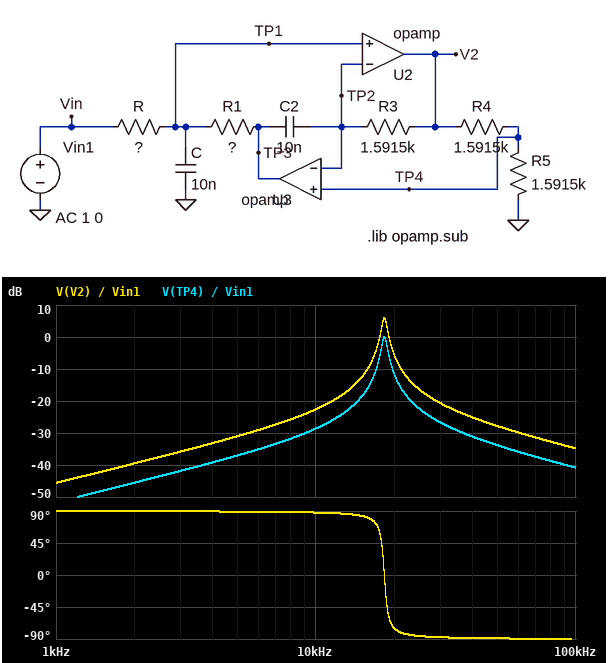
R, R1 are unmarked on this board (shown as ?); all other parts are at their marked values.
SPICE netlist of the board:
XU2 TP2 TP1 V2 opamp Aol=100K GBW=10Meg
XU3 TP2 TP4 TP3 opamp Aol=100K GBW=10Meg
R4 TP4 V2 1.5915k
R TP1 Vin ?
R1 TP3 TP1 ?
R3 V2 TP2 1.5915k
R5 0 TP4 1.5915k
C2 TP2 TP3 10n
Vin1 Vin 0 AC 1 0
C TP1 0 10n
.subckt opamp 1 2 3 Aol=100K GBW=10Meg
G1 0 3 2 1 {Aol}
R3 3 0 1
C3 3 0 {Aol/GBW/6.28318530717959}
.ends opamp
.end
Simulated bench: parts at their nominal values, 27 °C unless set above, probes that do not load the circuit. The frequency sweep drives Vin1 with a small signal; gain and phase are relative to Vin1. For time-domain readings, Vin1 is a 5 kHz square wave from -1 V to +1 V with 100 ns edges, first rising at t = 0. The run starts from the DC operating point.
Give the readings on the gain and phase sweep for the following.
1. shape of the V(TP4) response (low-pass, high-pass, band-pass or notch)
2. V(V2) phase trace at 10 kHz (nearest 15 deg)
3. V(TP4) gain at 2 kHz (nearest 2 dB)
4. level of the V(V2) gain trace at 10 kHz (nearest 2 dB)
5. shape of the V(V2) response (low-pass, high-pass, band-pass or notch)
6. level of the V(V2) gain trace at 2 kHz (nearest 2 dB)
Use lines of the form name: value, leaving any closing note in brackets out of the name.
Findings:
shape of the V(TP4) response: band-pass
V(V2) phase trace at 10 kHz: 90 deg
V(TP4) gain at 2 kHz: -46 dB
level of the V(V2) gain trace at 10 kHz: -22 dB
shape of the V(V2) response: band-pass
level of the V(V2) gain trace at 2 kHz: -40 dB
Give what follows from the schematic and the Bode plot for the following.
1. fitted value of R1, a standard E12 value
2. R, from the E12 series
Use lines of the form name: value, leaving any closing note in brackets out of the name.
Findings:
fitted value of R1, a standard E12 value: 470 Ω
R, from the E12 series: 18 kΩ
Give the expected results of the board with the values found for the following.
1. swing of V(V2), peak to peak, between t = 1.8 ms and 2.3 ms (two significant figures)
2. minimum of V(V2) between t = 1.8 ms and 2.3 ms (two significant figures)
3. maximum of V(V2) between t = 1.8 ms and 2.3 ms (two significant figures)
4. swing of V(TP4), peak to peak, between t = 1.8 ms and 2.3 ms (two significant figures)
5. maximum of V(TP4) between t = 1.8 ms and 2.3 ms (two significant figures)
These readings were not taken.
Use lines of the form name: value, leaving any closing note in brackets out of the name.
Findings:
swing of V(V2), peak to peak, between t = 1.8 ms and 2.3 ms: 250 mV
minimum of V(V2) between t = 1.8 ms and 2.3 ms: -120 mV
maximum of V(V2) between t = 1.8 ms and 2.3 ms: 120 mV
swing of V(TP4), peak to peak, between t = 1.8 ms and 2.3 ms: 120 mV
maximum of V(TP4) between t = 1.8 ms and 2.3 ms: 61 mV
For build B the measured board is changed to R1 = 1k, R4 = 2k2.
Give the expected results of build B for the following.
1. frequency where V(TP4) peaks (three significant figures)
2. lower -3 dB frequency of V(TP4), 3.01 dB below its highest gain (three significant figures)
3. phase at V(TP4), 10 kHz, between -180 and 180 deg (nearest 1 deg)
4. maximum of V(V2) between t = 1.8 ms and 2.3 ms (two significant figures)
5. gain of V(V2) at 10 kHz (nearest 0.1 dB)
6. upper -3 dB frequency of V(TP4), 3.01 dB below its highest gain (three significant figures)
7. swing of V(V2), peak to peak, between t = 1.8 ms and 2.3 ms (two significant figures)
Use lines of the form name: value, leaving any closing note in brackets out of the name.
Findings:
frequency where V(TP4) peaks: 14.8 kHz
lower -3 dB frequency of V(TP4), 3.01 dB below its highest gain: 14.4 kHz
phase at V(TP4), 10 kHz, between -180 and 180 deg: 86 deg
maximum of V(V2) between t = 1.8 ms and 2.3 ms: 1.0 V
gain of V(V2) at 10 kHz: -15.1 dB
upper -3 dB frequency of V(TP4), 3.01 dB below its highest gain: 15.2 kHz
swing of V(V2), peak to peak, between t = 1.8 ms and 2.3 ms: 2.0 V
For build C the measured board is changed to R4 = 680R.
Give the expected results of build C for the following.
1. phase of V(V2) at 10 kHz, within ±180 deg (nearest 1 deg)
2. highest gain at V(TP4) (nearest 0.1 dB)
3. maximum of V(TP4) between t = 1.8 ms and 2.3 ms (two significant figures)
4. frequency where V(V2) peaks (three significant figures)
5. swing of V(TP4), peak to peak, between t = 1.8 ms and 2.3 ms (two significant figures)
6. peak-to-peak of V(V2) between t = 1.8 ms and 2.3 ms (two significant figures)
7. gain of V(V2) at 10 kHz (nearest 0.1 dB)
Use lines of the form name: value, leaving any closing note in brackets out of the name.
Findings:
phase of V(V2) at 10 kHz, within ±180 deg: 78 deg
highest gain at V(TP4): -0.3 dB
maximum of V(TP4) between t = 1.8 ms and 2.3 ms: 95 mV
frequency where V(V2) peaks: 12.0 kHz
swing of V(TP4), peak to peak, between t = 1.8 ms and 2.3 ms: 190 mV
peak-to-peak of V(V2) between t = 1.8 ms and 2.3 ms: 270 mV
gain of V(V2) at 10 kHz: -11.0 dB
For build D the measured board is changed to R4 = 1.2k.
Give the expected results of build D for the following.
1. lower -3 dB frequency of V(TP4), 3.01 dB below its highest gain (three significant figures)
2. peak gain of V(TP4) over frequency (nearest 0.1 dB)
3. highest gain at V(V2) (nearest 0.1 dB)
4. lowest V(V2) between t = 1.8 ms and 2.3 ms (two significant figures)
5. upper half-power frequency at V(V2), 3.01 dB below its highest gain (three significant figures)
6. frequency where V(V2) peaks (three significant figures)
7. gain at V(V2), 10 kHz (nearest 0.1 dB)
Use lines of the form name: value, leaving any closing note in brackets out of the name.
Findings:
lower -3 dB frequency of V(TP4), 3.01 dB below its highest gain: 15.5 kHz
peak gain of V(TP4) over frequency: -0.2 dB
highest gain at V(V2): 4.7 dB
lowest V(V2) between t = 1.8 ms and 2.3 ms: -350 mV
upper half-power frequency at V(V2), 3.01 dB below its highest gain: 16.4 kHz
frequency where V(V2) peaks: 15.9 kHz
gain at V(V2), 10 kHz: -20.0 dB
